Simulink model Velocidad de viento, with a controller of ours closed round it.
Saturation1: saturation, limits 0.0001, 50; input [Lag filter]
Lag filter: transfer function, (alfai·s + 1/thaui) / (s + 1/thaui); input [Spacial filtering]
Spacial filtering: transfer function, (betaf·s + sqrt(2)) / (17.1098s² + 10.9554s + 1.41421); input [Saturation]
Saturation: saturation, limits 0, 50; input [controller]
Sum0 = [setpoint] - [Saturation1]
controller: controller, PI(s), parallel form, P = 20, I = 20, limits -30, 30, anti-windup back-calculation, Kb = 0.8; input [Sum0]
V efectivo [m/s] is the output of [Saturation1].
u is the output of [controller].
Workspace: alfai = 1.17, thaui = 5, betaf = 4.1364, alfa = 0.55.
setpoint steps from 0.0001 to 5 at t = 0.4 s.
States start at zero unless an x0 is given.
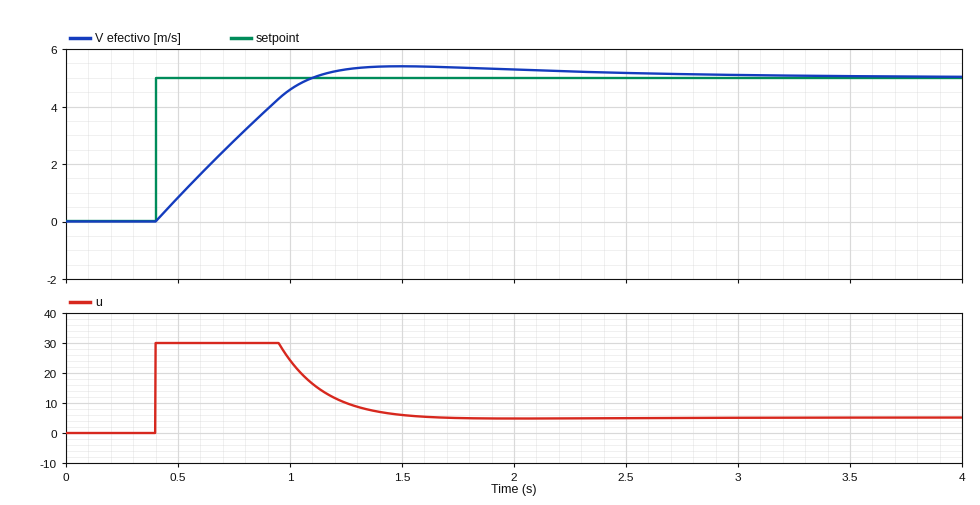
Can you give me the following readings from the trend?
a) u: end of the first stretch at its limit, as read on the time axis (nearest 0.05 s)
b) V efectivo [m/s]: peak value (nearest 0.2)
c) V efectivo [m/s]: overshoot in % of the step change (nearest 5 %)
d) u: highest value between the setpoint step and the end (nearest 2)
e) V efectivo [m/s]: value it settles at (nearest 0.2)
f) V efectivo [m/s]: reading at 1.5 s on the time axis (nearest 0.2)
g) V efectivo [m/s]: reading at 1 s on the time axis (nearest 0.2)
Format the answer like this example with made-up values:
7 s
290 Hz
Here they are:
0.95 s
5.4
10 %
30
5.0
5.4
4.6
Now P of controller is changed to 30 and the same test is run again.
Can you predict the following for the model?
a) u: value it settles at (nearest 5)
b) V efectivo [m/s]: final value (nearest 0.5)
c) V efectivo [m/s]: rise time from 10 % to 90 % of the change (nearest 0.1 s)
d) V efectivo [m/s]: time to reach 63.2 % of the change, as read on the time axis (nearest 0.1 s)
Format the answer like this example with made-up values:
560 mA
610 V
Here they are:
5
5.0
0.5 s
0.8 s
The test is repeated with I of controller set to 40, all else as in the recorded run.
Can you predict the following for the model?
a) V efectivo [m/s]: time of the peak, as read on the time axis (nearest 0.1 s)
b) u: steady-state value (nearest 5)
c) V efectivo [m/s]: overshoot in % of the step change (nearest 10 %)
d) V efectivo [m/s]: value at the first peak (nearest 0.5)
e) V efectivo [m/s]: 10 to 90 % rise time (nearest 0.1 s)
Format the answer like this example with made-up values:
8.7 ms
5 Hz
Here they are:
1.4 s
5
20 %
6.0
0.5 s
